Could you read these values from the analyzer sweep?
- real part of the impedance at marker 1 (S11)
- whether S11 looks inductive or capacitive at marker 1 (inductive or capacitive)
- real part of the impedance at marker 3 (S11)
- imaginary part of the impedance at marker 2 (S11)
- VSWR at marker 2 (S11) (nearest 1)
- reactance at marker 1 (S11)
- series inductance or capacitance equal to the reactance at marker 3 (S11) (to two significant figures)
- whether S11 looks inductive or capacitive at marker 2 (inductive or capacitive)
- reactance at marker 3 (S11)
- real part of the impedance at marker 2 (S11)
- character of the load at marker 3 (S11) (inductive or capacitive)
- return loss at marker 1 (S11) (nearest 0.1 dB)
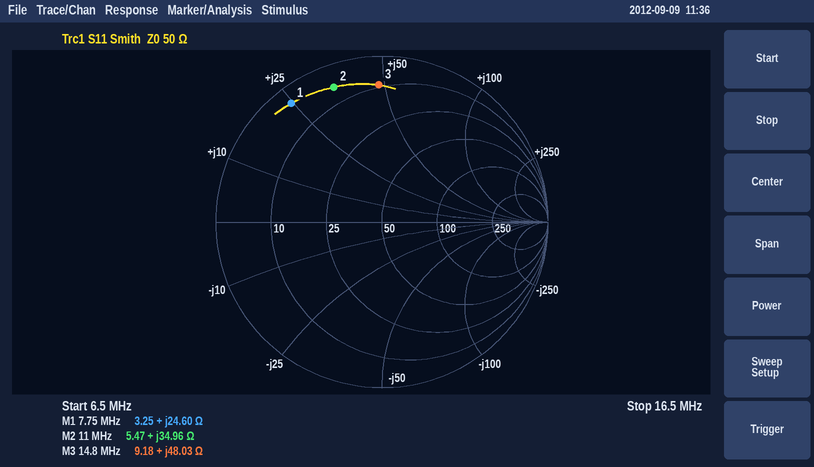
3.25 Ω
inductive
9.18 Ω
+34.96 Ω
14
+24.60 Ω
520 nH
inductive
+48.03 Ω
5.47 Ω
inductive
0.9 dB
